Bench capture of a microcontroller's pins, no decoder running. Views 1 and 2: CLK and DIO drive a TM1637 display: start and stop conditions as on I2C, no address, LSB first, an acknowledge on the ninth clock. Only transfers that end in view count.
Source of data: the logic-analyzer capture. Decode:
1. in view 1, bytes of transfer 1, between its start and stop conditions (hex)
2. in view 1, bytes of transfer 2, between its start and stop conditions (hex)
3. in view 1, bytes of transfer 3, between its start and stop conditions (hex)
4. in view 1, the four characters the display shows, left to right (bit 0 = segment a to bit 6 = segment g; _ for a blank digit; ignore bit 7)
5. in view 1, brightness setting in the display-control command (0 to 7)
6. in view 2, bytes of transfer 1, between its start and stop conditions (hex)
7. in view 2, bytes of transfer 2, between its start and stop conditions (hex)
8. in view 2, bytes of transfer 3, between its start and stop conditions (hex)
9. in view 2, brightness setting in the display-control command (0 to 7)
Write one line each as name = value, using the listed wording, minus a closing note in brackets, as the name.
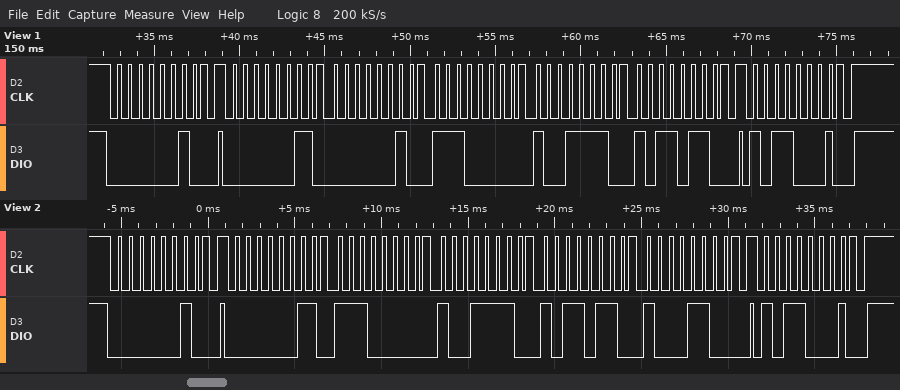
in view 1, bytes of transfer 1, between its start and stop conditions = 40
in view 1, bytes of transfer 2, between its start and stop conditions = C0 40 07 79 6D
in view 1, bytes of transfer 3, between its start and stop conditions = 8D
in view 1, the four characters the display shows, left to right = -7E5
in view 1, brightness setting in the display-control command = 5
in view 2, bytes of transfer 1, between its start and stop conditions = 40
in view 2, bytes of transfer 2, between its start and stop conditions = C0 07 79 6D 31
in view 2, bytes of transfer 3, between its start and stop conditions = 8D
in view 2, brightness setting in the display-control command = 5
